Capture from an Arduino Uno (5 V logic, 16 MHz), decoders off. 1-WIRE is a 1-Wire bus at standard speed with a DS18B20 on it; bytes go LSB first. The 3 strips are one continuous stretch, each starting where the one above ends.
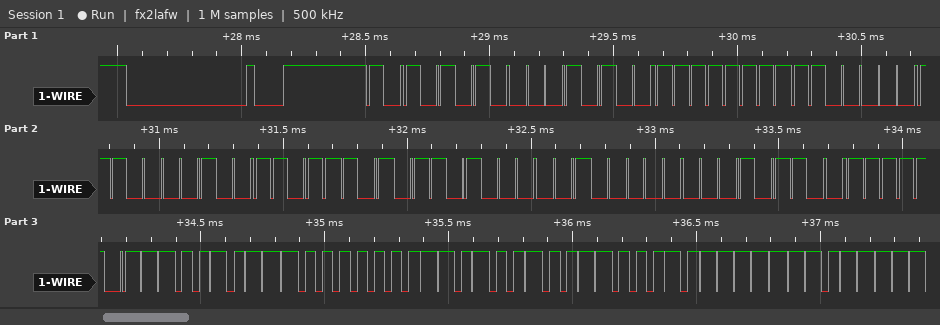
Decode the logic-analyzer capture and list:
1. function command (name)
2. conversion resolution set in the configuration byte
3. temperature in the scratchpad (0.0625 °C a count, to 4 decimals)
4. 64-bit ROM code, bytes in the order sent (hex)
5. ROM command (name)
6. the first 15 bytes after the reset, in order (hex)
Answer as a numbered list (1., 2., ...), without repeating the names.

1. Read Scratchpad
2. 12 bits
3. 29.1875 °C
4. 28 FF 83 21 BB 16 04 68
5. Match ROM
6. 55 28 FF 83 21 BB 16 04 68 BE D3 01 4B 46 7F
